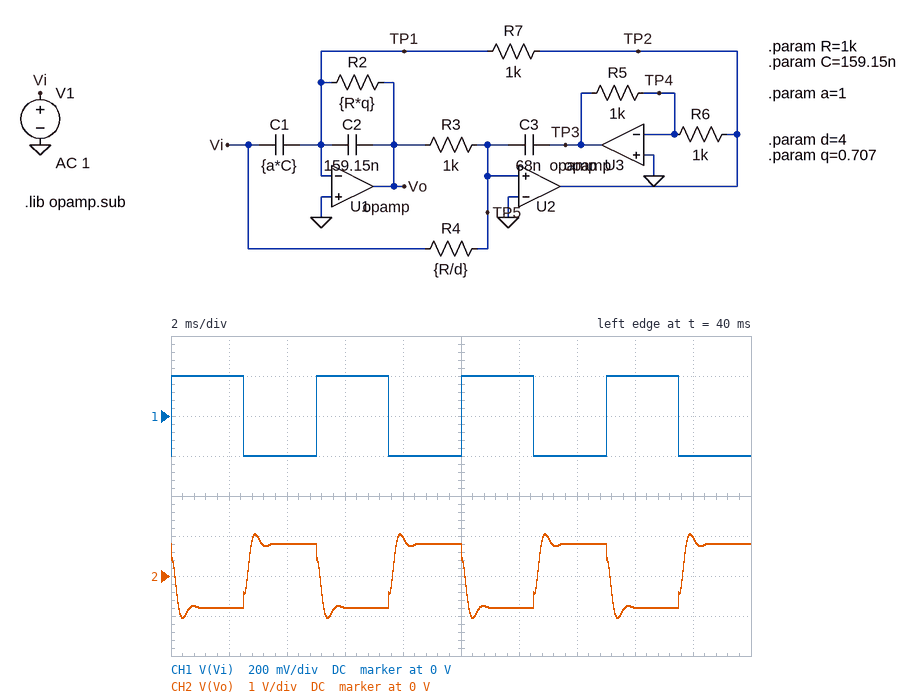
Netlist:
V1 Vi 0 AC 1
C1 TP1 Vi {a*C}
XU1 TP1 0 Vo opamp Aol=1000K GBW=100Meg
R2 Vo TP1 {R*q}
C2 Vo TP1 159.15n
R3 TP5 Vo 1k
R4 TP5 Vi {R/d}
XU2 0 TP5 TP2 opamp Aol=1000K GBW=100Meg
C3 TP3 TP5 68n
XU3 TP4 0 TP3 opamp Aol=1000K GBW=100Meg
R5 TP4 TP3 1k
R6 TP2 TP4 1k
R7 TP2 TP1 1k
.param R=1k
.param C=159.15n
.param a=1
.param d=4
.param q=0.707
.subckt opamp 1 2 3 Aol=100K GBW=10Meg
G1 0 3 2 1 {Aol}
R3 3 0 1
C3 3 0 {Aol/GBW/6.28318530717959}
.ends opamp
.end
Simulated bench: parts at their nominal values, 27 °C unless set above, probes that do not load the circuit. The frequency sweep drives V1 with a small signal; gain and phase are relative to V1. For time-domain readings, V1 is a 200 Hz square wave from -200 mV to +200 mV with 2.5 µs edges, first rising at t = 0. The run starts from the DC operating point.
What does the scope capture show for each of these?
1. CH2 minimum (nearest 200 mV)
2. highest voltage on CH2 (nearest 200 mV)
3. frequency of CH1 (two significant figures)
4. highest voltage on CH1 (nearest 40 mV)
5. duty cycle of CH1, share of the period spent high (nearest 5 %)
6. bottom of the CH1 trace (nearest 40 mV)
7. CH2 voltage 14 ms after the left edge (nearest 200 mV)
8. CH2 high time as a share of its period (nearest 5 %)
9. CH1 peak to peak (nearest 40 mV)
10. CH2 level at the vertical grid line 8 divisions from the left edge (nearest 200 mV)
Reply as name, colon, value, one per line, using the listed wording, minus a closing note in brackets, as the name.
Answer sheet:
CH2 minimum: -1.0 V
highest voltage on CH2: 1.0 V
frequency of CH1: 200 Hz
highest voltage on CH1: 200 mV
duty cycle of CH1, share of the period spent high: 50 %
bottom of the CH1 trace: -200 mV
CH2 voltage 14 ms after the left edge: 800 mV
CH2 high time as a share of its period: 50 %
CH1 peak to peak: 400 mV
CH2 level at the vertical grid line 8 divisions from the left edge: -800 mV
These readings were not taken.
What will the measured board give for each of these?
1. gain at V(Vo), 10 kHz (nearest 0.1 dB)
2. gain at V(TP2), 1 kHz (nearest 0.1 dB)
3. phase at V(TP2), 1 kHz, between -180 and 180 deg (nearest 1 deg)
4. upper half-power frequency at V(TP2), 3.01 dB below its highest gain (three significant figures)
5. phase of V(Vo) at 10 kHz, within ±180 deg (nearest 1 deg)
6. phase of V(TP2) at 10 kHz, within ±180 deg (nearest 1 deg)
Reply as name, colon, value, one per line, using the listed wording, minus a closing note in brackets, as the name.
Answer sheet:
gain at V(Vo), 10 kHz: -0.7 dB
gain at V(TP2), 1 kHz: 17.7 dB
phase at V(TP2), 1 kHz, between -180 and 180 deg: -19 deg
upper half-power frequency at V(TP2), 3.01 dB below its highest gain: 2.01 kHz
phase of V(Vo) at 10 kHz, within ±180 deg: -172 deg
phase of V(TP2) at 10 kHz, within ±180 deg: -92 deg
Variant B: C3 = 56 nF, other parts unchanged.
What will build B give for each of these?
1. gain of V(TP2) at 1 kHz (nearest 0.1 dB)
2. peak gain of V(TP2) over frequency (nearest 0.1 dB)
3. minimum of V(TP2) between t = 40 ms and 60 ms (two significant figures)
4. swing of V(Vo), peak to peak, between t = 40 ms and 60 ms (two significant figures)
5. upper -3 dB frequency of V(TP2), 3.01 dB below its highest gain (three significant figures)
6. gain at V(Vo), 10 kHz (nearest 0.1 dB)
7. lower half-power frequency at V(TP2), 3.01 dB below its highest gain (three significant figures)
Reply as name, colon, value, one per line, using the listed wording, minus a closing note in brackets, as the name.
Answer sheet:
gain of V(TP2) at 1 kHz: 17.9 dB
peak gain of V(TP2) over frequency: 19.4 dB
minimum of V(TP2) between t = 40 ms and 60 ms: -2.0 V
swing of V(Vo), peak to peak, between t = 40 ms and 60 ms: 2.2 V
upper -3 dB frequency of V(TP2), 3.01 dB below its highest gain: 2.22 kHz
gain at V(Vo), 10 kHz: -0.9 dB
lower half-power frequency at V(TP2), 3.01 dB below its highest gain: 658 Hz
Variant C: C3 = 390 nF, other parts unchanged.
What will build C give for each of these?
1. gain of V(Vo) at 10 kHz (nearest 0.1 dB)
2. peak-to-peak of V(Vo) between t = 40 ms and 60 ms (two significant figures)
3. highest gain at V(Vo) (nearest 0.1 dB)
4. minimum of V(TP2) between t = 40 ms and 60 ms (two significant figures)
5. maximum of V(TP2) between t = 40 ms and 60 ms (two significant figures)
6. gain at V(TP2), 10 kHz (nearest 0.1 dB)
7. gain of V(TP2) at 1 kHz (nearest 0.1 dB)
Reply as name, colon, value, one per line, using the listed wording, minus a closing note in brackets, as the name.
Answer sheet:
gain of V(Vo) at 10 kHz: -0.2 dB
peak-to-peak of V(Vo) between t = 40 ms and 60 ms: 1.6 V
highest gain at V(Vo): 12.0 dB
minimum of V(TP2) between t = 40 ms and 60 ms: -1.1 V
maximum of V(TP2) between t = 40 ms and 60 ms: 1.1 V
gain at V(TP2), 10 kHz: -18.1 dB
gain of V(TP2) at 1 kHz: 4.6 dB
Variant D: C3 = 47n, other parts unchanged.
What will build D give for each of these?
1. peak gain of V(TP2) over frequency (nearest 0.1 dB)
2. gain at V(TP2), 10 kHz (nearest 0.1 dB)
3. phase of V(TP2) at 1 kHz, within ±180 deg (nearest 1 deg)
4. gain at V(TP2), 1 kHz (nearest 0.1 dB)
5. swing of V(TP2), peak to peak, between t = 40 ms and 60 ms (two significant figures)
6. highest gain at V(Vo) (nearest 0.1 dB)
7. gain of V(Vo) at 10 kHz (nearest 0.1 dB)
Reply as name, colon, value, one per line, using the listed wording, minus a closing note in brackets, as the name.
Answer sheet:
peak gain of V(TP2) over frequency: 20.4 dB
gain at V(TP2), 10 kHz: 0.5 dB
phase of V(TP2) at 1 kHz, within ±180 deg: -3 deg
gain at V(TP2), 1 kHz: 17.9 dB
swing of V(TP2), peak to peak, between t = 40 ms and 60 ms: 4.3 V
highest gain at V(Vo): 13.5 dB
gain of V(Vo) at 10 kHz: -1.1 dB
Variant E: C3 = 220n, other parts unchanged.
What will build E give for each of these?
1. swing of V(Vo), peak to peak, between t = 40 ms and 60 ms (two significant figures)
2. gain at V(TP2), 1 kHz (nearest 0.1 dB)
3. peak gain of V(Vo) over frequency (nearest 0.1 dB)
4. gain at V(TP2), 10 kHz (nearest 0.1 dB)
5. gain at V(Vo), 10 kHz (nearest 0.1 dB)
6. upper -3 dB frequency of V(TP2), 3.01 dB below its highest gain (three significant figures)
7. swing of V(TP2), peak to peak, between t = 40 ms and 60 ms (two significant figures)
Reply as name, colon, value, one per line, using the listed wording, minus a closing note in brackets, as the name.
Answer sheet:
swing of V(Vo), peak to peak, between t = 40 ms and 60 ms: 1.6 V
gain at V(TP2), 1 kHz: 10.1 dB
peak gain of V(Vo) over frequency: 12.0 dB
gain at V(TP2), 10 kHz: -13.1 dB
gain at V(Vo), 10 kHz: -0.3 dB
upper -3 dB frequency of V(TP2), 3.01 dB below its highest gain: 778 Hz
swing of V(TP2), peak to peak, between t = 40 ms and 60 ms: 2.3 V
